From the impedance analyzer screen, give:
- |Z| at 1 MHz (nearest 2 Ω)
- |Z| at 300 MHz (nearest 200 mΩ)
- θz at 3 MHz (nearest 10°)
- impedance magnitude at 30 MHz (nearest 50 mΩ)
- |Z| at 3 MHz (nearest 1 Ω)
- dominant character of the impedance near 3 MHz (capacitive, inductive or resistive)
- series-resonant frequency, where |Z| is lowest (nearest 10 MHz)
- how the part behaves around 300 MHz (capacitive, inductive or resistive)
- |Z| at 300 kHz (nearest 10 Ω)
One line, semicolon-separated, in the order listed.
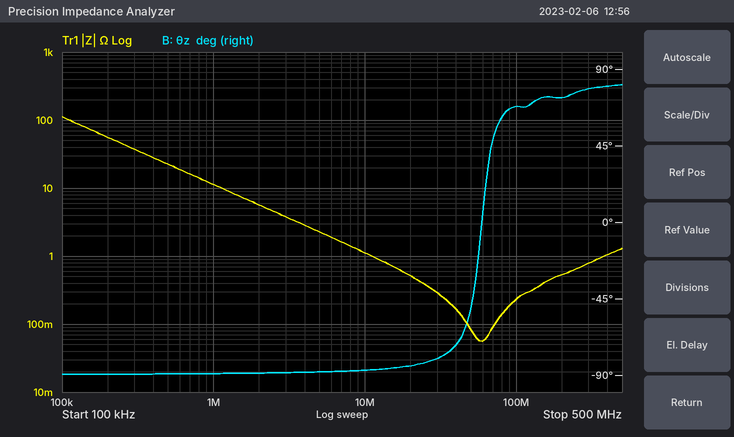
12 Ω; 800 mΩ; -90°; 300 mΩ; 4 Ω; capacitive; 60 MHz; inductive; 40 Ω
